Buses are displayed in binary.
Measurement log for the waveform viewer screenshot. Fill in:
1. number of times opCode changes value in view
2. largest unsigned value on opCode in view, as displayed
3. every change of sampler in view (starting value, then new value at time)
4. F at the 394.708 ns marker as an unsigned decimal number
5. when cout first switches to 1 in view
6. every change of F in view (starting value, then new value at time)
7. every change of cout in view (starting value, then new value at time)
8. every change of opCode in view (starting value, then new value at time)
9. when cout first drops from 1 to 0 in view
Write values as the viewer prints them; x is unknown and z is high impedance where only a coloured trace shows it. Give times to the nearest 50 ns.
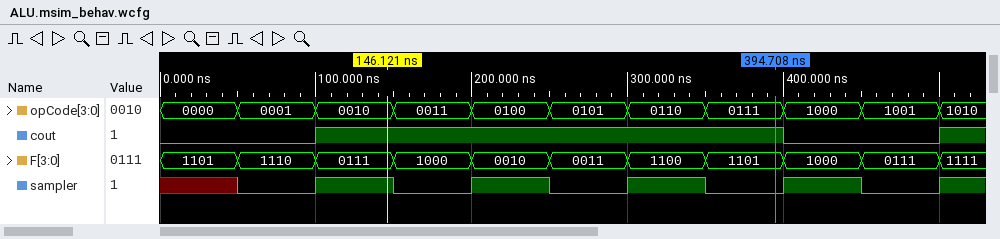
10
1010
x, 0 at 50 ns, 1 at 100 ns, 0 at 150 ns, 1 at 200 ns, 0 at 250 ns, 1 at 300 ns, 0 at 350 ns, 1 at 400 ns, 0 at 450 ns, 1 at 500 ns
13
100 ns
1101, 1110 at 50 ns, 0111 at 100 ns, 1000 at 150 ns, 0010 at 200 ns, 0011 at 250 ns, 1100 at 300 ns, 1101 at 350 ns, 1000 at 400 ns, 0111 at 450 ns, 1111 at 500 ns
0, 1 at 100 ns, 0 at 400 ns, 1 at 500 ns
0000, 0001 at 50 ns, 0010 at 100 ns, 0011 at 150 ns, 0100 at 200 ns, 0101 at 250 ns, 0110 at 300 ns, 0111 at 350 ns, 1000 at 400 ns, 1001 at 450 ns, 1010 at 500 ns
400 ns
